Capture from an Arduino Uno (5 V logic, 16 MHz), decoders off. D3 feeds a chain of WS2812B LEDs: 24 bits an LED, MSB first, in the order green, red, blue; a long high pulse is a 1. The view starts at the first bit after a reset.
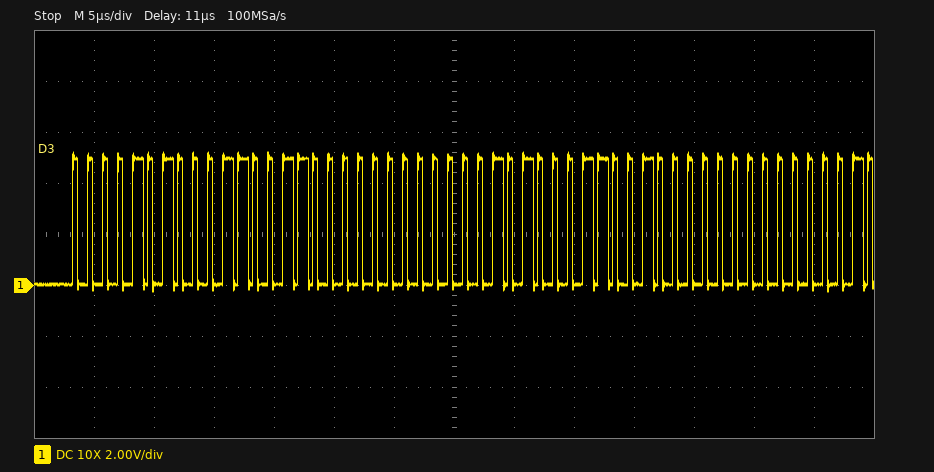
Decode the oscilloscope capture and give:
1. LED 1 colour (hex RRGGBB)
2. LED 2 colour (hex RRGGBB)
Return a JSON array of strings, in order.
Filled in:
["#330A00", "#320A00"]
